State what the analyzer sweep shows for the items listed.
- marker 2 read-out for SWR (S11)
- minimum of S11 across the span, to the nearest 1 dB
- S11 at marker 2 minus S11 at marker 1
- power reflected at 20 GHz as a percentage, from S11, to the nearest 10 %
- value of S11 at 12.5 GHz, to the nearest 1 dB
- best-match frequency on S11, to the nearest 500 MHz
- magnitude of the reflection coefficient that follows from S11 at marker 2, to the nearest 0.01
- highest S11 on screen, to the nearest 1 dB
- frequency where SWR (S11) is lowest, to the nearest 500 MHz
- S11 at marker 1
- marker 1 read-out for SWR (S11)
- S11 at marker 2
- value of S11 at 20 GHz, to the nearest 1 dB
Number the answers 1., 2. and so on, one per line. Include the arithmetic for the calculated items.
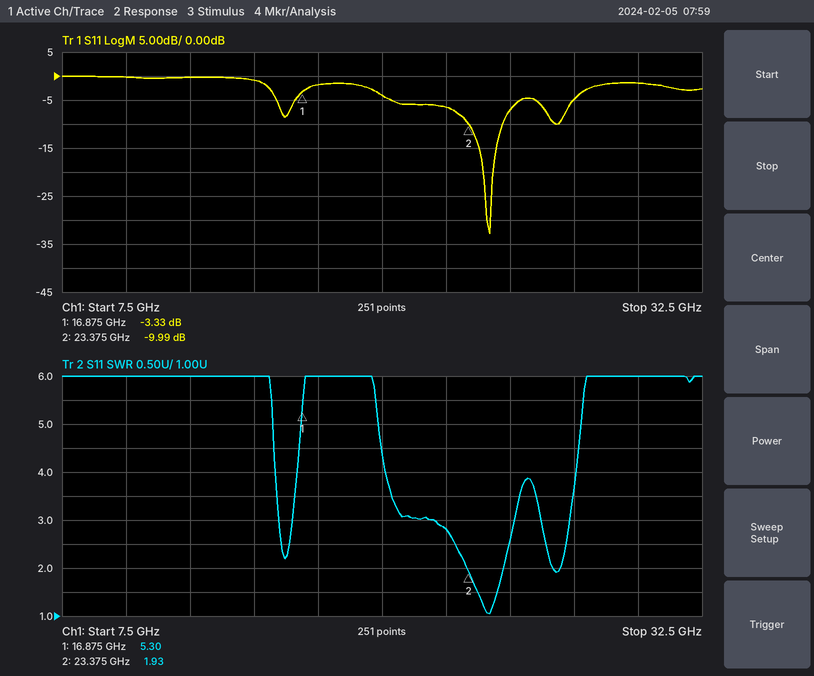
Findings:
1. 1.93
2. -33 dB
3. -9.99 − (-3.33) = -6.66 dB
4. 10^(-4/10) ≈ 40 %
5. 0 dB
6. 24.0 GHz
7. 10^(-9.99/20) ≈ 0.32
8. 0 dB
9. 24.0 GHz
10. -3.33 dB
11. 5.30
12. -9.99 dB
13. -4 dB
